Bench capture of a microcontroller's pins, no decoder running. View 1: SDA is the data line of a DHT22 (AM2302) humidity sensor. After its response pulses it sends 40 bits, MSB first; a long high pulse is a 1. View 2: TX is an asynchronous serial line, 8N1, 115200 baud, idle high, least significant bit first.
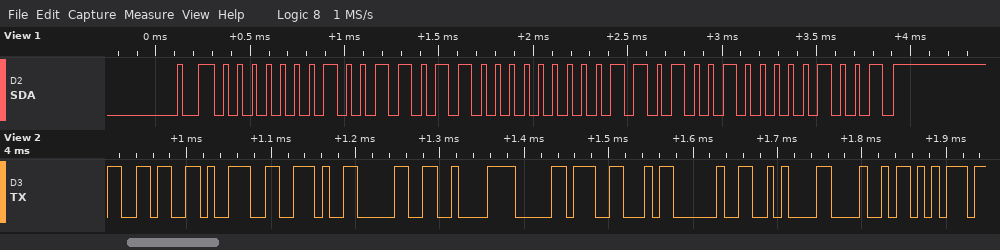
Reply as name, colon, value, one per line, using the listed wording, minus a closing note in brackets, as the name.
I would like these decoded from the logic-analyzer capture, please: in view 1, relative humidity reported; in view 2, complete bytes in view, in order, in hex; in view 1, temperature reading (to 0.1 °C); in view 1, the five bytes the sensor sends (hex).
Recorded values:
in view 1, relative humidity reported: 31.0 %
in view 2, complete bytes in view, in order, in hex: 0x36 0x39 0x2E 0x30 0xC2 0xB0 0x46 0x20 0x0A 0x48 0x75
in view 1, temperature reading: 21.0 °C
in view 1, the five bytes the sensor sends: 01 36 00 D2 09
